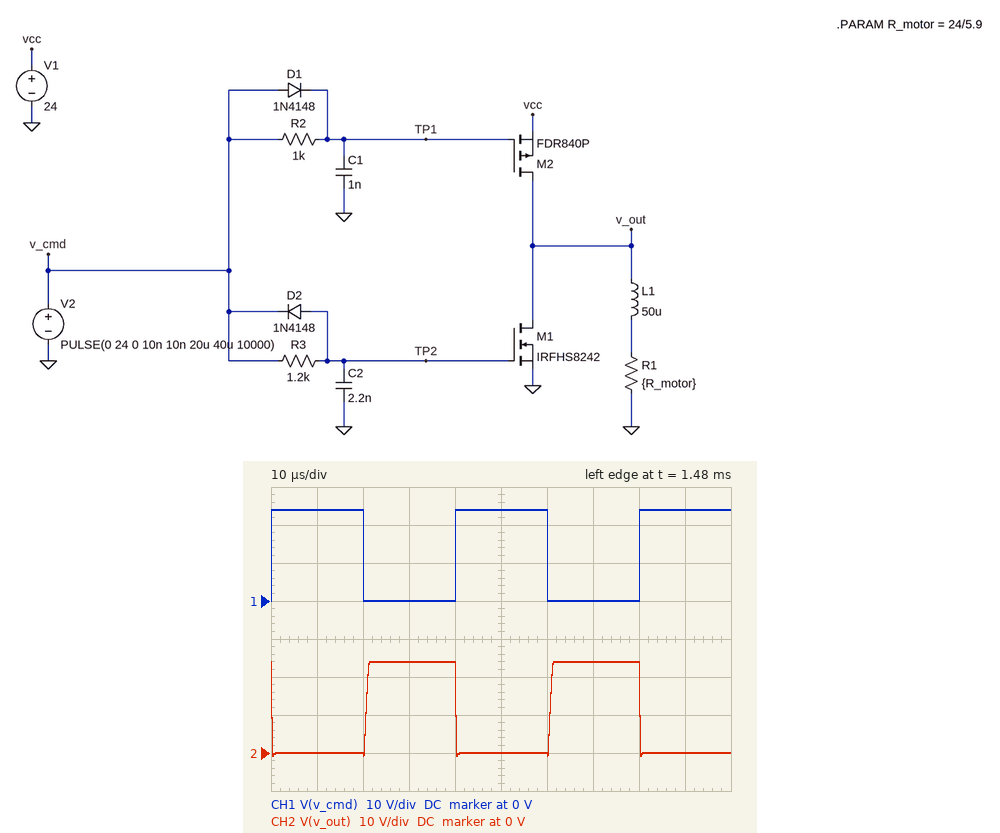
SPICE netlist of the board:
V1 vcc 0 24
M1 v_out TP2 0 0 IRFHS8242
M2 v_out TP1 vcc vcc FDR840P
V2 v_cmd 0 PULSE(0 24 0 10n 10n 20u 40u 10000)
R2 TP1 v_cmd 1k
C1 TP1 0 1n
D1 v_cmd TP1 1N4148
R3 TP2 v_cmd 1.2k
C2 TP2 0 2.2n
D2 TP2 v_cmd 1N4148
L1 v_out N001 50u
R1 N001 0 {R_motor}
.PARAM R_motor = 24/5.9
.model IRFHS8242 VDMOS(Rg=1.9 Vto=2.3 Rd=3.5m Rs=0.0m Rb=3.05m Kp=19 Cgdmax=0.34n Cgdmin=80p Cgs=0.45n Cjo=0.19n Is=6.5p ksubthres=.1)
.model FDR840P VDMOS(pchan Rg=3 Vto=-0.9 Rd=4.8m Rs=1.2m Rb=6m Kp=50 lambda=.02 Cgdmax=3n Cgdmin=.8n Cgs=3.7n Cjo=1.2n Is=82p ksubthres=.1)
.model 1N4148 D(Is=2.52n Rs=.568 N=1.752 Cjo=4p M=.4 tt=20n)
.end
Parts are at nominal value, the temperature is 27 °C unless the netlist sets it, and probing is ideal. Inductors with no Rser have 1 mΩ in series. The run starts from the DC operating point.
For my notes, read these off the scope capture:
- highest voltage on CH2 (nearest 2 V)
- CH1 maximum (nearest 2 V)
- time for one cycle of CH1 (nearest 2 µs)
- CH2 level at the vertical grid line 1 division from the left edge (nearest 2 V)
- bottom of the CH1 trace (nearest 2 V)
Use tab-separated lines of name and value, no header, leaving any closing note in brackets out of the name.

highest voltage on CH2	24 V
CH1 maximum	24 V
time for one cycle of CH1	40 µs
CH2 level at the vertical grid line 1 division from the left edge	0 V
bottom of the CH1 trace	0 V
